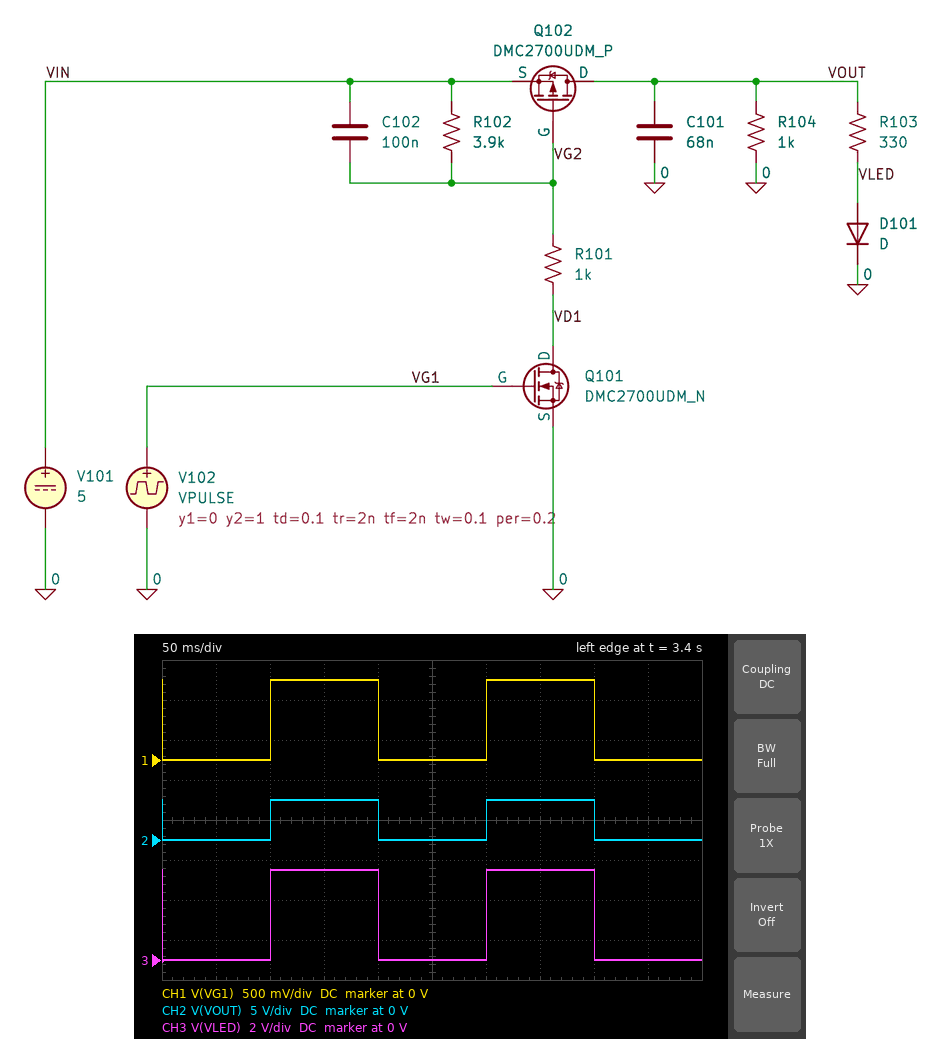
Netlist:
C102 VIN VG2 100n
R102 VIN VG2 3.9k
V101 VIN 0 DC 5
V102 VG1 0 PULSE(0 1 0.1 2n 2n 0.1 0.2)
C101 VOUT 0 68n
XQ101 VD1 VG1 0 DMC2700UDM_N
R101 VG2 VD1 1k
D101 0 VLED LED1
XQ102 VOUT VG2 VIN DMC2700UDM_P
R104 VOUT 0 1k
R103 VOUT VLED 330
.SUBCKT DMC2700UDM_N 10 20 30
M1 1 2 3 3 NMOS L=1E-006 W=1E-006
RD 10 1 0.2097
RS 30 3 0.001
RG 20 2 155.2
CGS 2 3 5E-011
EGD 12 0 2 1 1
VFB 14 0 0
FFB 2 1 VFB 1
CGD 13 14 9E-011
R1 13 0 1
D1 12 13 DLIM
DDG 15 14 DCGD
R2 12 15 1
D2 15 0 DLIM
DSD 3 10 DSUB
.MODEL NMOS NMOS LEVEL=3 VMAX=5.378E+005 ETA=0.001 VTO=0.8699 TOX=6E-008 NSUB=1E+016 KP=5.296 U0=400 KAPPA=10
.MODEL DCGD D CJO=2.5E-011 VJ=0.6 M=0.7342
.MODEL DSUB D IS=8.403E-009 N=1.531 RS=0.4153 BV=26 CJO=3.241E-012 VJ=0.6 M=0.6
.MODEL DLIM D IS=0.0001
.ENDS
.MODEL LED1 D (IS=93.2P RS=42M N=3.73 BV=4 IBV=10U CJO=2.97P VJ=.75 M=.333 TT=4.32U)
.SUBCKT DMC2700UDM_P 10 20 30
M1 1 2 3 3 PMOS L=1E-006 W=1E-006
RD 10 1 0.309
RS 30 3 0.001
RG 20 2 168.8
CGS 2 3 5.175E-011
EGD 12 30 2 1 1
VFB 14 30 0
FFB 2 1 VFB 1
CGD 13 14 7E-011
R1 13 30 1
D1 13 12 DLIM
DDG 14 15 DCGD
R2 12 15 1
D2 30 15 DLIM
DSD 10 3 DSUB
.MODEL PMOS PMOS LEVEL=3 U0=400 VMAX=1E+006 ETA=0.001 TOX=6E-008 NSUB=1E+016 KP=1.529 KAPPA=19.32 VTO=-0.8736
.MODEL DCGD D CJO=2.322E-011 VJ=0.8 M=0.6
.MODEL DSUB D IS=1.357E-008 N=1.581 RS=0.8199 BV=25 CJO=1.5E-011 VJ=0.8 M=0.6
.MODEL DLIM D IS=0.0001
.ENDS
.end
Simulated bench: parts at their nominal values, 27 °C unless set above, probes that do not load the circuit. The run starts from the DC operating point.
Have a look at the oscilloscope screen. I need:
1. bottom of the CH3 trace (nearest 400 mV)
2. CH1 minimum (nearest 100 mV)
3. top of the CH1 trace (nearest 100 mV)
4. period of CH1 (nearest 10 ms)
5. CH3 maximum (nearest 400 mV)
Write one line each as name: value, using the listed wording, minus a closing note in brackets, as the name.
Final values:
bottom of the CH3 trace: 0 V
CH1 minimum: 0 V
top of the CH1 trace: 1.0 V
period of CH1: 200 ms
CH3 maximum: 4.4 V
